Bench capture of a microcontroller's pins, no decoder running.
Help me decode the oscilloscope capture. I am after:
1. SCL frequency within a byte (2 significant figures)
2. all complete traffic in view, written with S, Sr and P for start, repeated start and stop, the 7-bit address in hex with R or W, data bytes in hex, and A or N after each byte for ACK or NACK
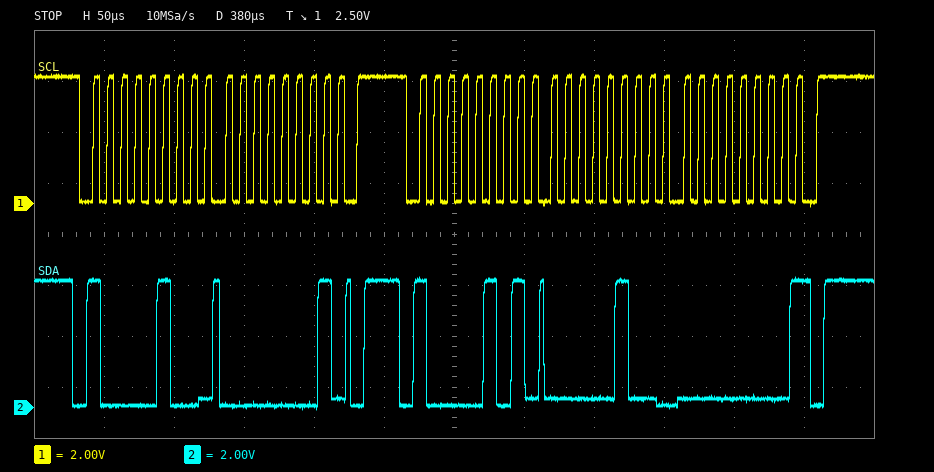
100 kHz
S 42W A 01 A P S 42R A 04 A 00 N P
